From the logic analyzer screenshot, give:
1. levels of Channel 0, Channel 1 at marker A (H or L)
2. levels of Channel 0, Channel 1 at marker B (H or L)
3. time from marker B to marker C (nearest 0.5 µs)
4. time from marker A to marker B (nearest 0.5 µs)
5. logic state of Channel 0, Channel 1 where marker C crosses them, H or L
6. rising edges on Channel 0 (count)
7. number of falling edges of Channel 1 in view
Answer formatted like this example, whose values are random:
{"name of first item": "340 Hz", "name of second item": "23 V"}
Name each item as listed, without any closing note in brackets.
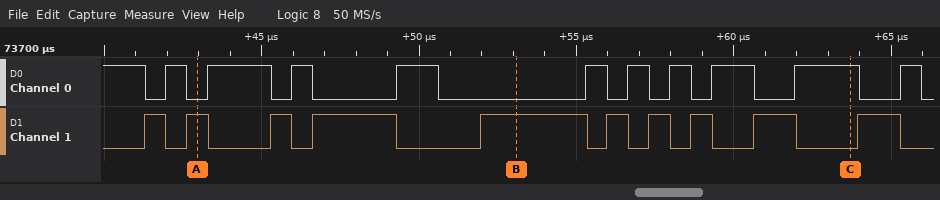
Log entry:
{"levels of Channel 0, Channel 1 at marker A": "Channel 0=L, Channel 1=H", "levels of Channel 0, Channel 1 at marker B": "Channel 0=L, Channel 1=H", "time from marker B to marker C": "10.5 µs", "time from marker A to marker B": "10 µs", "logic state of Channel 0, Channel 1 where marker C crosses them, H or L": "Channel 0=H, Channel 1=L", "rising edges on Channel 0": "10", "number of falling edges of Channel 1 in view": "10"}
